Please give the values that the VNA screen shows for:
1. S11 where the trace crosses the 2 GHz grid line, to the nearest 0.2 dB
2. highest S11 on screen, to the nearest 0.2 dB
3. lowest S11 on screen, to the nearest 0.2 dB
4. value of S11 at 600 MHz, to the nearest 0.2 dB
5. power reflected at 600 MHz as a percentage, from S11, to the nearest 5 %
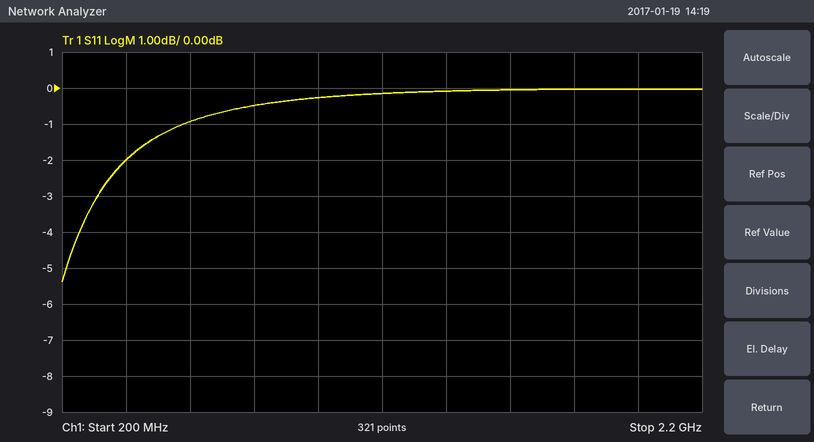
0.0 dB
0.0 dB
-5.4 dB
-1.0 dB
80 %
